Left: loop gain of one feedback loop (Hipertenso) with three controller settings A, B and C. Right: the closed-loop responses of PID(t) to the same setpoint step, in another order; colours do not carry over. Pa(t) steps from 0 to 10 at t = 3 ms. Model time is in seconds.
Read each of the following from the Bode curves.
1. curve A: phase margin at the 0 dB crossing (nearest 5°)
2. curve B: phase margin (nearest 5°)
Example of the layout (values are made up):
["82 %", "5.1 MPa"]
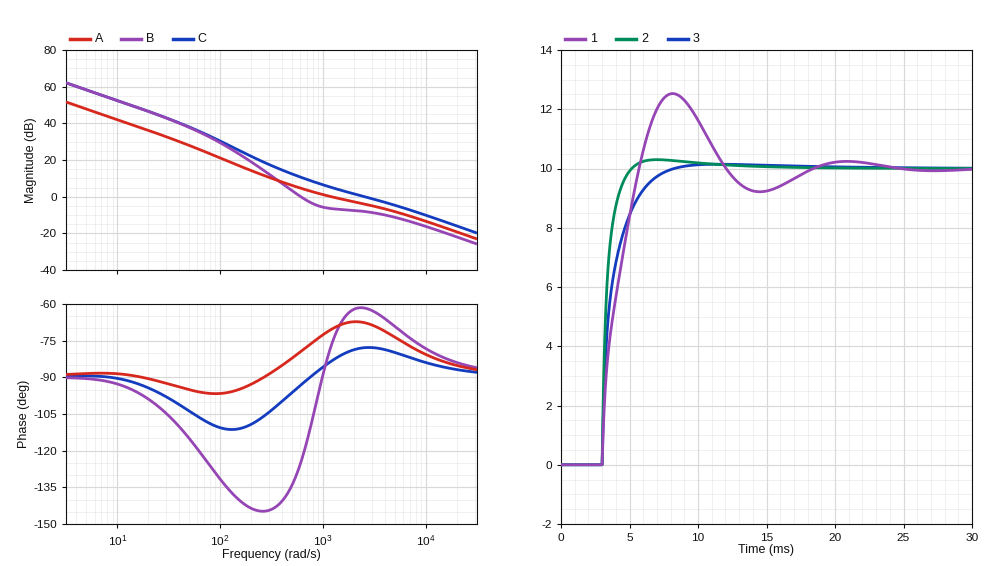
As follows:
["110°", "55°"]
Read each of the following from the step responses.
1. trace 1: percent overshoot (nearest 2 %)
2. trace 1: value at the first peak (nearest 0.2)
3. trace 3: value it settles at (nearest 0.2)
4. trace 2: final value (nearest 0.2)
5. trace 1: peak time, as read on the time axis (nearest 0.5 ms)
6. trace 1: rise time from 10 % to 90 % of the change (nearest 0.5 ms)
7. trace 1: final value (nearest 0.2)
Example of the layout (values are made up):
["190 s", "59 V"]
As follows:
["26 %", "12.6", "10.0", "10.0", "8.0 ms", "2.0 ms", "10.0"]
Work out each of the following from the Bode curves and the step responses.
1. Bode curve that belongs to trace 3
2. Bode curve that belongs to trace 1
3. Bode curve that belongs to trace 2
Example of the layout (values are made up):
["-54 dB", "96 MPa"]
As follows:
["A", "B", "C"]
